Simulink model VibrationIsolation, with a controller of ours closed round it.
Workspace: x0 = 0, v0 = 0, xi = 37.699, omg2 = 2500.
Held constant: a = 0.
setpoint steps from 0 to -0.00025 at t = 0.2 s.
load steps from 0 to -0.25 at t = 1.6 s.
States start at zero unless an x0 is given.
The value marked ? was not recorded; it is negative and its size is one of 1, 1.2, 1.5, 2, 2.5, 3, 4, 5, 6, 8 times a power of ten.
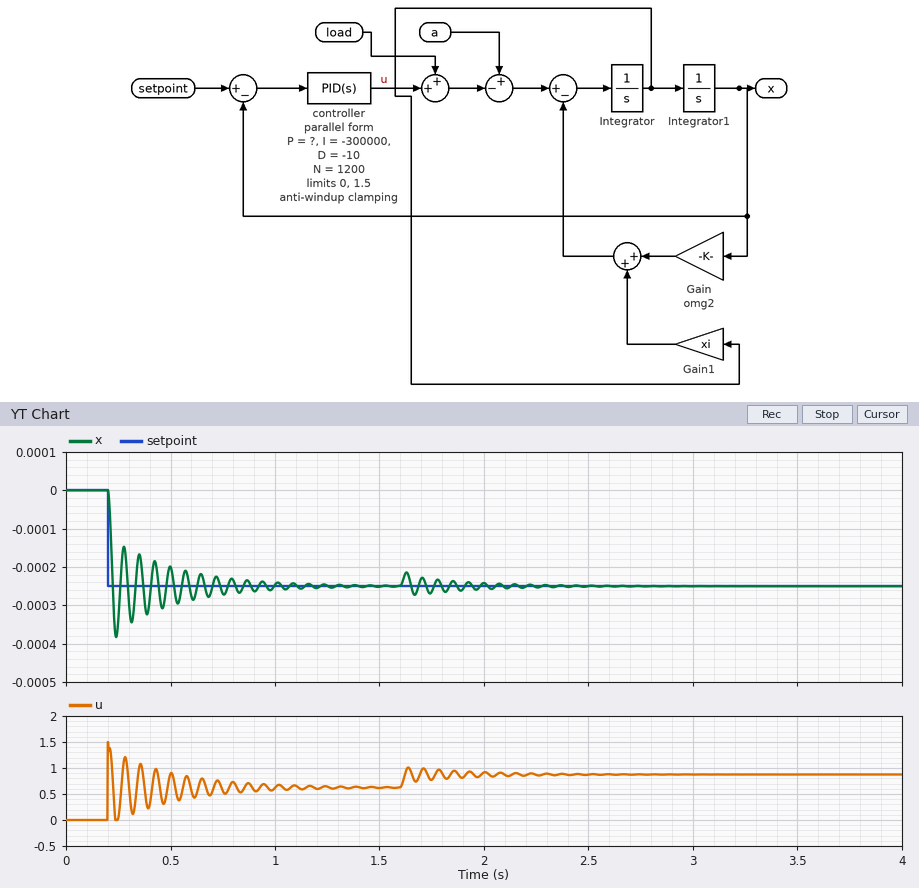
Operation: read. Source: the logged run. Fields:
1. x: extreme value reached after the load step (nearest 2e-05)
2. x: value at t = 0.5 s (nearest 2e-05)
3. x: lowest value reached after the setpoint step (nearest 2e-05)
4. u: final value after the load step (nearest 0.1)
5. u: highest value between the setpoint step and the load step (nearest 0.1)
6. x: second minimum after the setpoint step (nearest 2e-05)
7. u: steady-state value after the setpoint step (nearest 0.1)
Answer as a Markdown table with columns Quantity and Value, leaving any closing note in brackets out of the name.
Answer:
| Quantity | Value |
|---|---|
| x: extreme value reached after the load step | -0.00022 |
| x: value at t = 0.5 s | -0.00020 |
| x: lowest value reached after the setpoint step | -0.00038 |
| u: final value after the load step | 0.9 |
| u: highest value between the setpoint step and the load step | 1.5 |
| x: second minimum after the setpoint step | -0.00034 |
| u: steady-state value after the setpoint step | 0.6 |
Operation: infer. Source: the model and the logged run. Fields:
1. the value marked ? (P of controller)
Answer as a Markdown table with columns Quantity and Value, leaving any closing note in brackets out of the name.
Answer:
| Quantity | Value |
|---|---|
| the value marked ? | -5000 |
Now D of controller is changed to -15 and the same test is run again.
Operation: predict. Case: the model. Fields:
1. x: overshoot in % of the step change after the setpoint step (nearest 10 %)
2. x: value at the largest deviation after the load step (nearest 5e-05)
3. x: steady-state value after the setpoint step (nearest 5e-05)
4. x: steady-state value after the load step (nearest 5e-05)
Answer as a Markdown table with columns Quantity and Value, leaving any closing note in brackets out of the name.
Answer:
| Quantity | Value |
|---|---|
| x: overshoot in % of the step change after the setpoint step | 50 % |
| x: value at the largest deviation after the load step | -0.00020 |
| x: steady-state value after the setpoint step | -0.00025 |
| x: steady-state value after the load step | -0.00025 |
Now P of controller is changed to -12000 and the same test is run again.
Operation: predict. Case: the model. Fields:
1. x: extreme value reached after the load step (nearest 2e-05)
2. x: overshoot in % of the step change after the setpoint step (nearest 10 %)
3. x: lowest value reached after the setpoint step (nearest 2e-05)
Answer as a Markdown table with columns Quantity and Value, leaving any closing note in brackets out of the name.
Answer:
| Quantity | Value |
|---|---|
| x: extreme value reached after the load step | -0.00022 |
| x: overshoot in % of the step change after the setpoint step | 30 % |
| x: lowest value reached after the setpoint step | -0.00032 |
